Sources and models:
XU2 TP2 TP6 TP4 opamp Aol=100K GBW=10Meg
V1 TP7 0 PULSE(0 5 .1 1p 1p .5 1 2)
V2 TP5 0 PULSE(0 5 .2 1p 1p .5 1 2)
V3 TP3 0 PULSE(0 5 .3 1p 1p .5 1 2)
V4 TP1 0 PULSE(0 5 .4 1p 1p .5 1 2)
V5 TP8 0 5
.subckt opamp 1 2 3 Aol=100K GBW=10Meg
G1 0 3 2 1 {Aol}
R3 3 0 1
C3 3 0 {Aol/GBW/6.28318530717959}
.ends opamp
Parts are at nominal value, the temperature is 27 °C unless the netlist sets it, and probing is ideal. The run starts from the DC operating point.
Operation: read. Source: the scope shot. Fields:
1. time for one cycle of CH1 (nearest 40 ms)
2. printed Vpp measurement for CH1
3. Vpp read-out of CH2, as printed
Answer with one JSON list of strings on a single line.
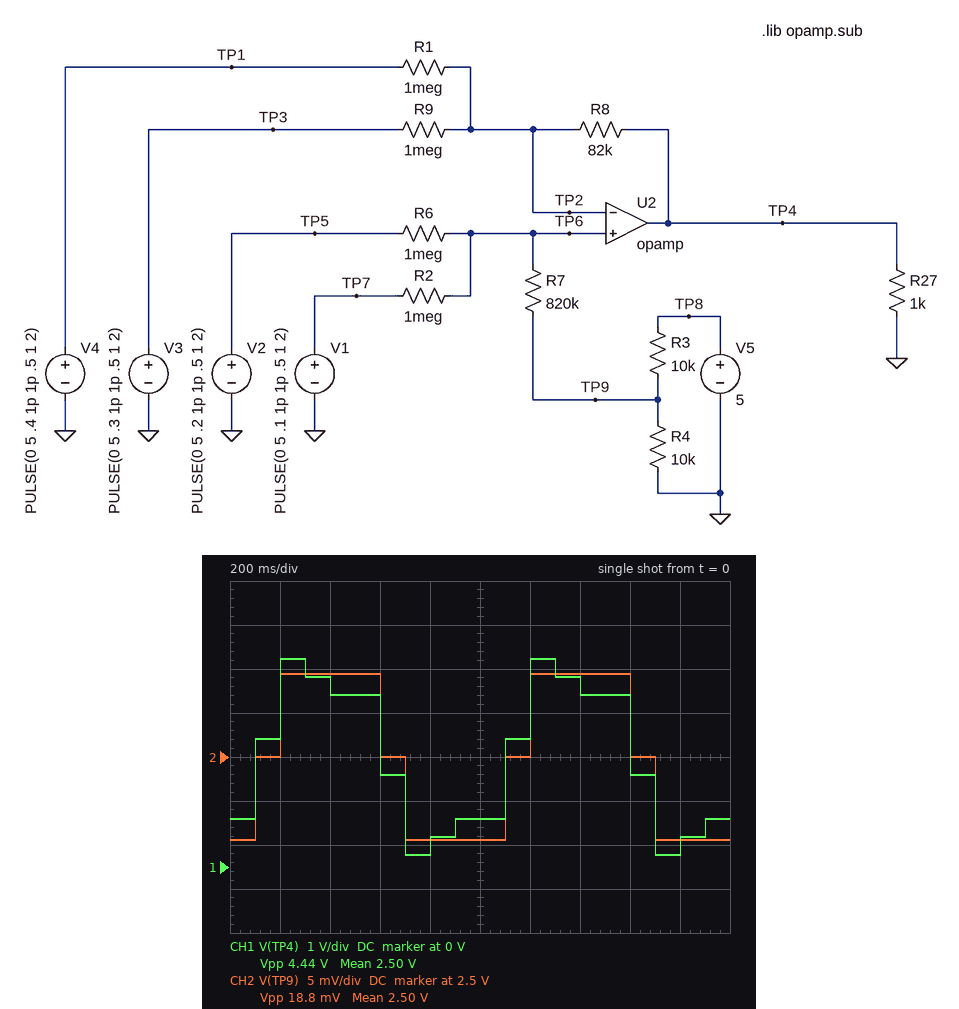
["1.00 s", "4.44 V", "18.8 mV"]
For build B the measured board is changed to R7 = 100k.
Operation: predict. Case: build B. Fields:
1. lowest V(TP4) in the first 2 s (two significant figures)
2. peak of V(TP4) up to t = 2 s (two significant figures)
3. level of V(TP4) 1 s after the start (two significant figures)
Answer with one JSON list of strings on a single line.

["1.6 V", "3.4 V", "2.4 V"]
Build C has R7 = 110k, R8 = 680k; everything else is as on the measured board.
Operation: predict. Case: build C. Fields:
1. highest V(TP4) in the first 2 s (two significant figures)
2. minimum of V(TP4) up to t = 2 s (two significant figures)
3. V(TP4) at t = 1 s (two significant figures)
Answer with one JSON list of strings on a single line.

["7.0 V", "-2.0 V", "4.8 V"]
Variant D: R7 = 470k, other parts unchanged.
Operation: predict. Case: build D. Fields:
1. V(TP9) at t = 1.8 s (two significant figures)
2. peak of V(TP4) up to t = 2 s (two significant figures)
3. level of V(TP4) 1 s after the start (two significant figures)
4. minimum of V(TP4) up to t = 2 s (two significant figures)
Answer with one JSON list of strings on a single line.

["2.5 V", "4.3 V", "1.5 V", "670 mV"]
